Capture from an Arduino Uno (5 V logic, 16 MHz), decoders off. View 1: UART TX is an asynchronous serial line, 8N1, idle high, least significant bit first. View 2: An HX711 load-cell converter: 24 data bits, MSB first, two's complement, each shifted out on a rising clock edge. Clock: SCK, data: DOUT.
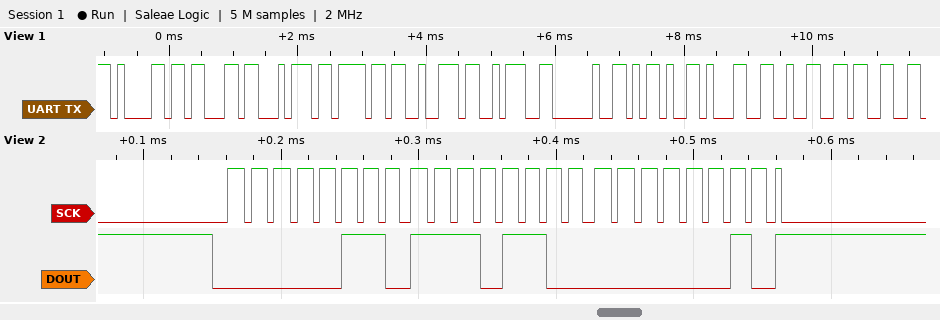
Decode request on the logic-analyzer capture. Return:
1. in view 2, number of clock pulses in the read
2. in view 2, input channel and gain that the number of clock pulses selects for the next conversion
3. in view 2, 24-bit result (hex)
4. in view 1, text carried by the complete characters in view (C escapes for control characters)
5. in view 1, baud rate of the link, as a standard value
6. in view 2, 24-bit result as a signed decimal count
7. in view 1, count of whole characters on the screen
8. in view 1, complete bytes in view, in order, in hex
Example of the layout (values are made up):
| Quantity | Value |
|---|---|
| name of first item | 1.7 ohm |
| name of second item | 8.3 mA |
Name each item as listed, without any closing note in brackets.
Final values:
| Quantity | Value |
|---|---|
| in view 2, number of clock pulses in the read | 25 |
| in view 2, input channel and gain that the number of clock pulses selects for the next conversion | channel A, gain 128 |
| in view 2, 24-bit result | 0x06EC02 |
| in view 1, text carried by the complete characters in view | "actor: -123" |
| in view 1, baud rate of the link, as a standard value | 9600 baud |
| in view 2, 24-bit result as a signed decimal count | 453634 |
| in view 1, count of whole characters on the screen | 11 |
| in view 1, complete bytes in view, in order, in hex | 61 63 74 6F 72 3A 20 2D 31 32 33 |
